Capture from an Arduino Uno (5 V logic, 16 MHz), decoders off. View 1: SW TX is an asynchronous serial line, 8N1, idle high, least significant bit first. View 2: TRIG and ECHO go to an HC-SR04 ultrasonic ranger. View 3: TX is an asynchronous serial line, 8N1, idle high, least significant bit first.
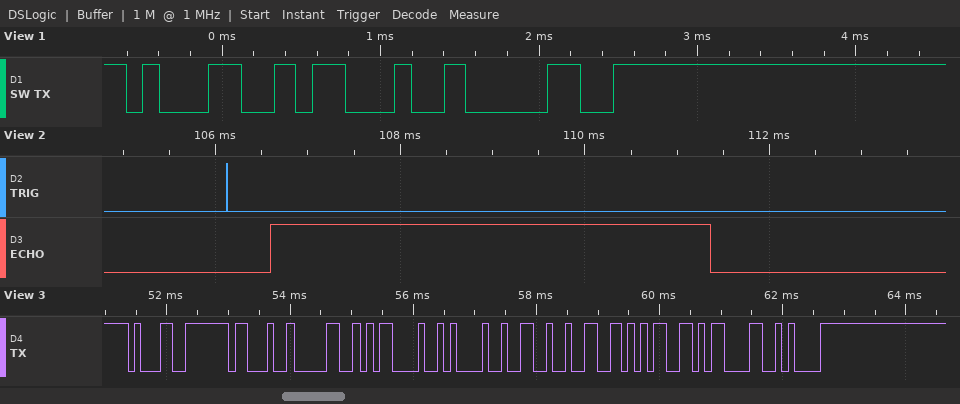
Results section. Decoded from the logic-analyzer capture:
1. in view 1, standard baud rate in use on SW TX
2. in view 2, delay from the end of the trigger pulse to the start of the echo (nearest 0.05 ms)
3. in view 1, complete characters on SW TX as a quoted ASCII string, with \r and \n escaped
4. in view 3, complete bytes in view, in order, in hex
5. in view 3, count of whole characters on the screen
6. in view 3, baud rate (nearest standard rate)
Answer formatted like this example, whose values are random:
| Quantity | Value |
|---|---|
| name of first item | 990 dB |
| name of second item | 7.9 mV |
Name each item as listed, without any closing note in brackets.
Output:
| Quantity | Value |
|---|---|
| in view 1, standard baud rate in use on SW TX | 9600 baud |
| in view 2, delay from the end of the trigger pulse to the start of the echo | 0.45 ms |
| in view 1, complete characters on SW TX as a quoted ASCII string, with \r and \n escaped | "1#0" |
| in view 3, complete bytes in view, in order, in hex | 31 23 30 0D 0A 32 32 35 0D 0A |
| in view 3, count of whole characters on the screen | 10 |
| in view 3, baud rate | 9600 baud |
